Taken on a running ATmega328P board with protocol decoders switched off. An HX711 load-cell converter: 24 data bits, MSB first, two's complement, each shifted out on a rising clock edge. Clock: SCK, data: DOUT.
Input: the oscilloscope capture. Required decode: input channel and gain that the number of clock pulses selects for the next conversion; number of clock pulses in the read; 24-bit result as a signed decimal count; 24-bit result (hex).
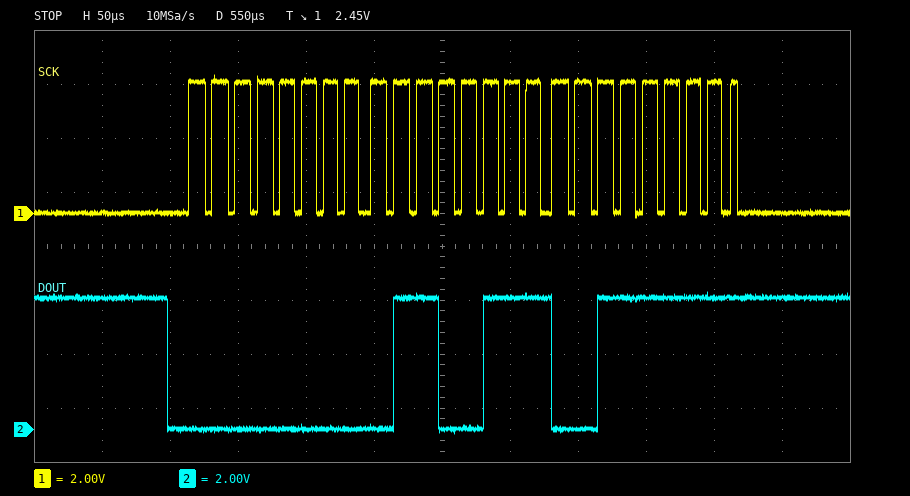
channel A, gain 128
25
26431
0x00673F
